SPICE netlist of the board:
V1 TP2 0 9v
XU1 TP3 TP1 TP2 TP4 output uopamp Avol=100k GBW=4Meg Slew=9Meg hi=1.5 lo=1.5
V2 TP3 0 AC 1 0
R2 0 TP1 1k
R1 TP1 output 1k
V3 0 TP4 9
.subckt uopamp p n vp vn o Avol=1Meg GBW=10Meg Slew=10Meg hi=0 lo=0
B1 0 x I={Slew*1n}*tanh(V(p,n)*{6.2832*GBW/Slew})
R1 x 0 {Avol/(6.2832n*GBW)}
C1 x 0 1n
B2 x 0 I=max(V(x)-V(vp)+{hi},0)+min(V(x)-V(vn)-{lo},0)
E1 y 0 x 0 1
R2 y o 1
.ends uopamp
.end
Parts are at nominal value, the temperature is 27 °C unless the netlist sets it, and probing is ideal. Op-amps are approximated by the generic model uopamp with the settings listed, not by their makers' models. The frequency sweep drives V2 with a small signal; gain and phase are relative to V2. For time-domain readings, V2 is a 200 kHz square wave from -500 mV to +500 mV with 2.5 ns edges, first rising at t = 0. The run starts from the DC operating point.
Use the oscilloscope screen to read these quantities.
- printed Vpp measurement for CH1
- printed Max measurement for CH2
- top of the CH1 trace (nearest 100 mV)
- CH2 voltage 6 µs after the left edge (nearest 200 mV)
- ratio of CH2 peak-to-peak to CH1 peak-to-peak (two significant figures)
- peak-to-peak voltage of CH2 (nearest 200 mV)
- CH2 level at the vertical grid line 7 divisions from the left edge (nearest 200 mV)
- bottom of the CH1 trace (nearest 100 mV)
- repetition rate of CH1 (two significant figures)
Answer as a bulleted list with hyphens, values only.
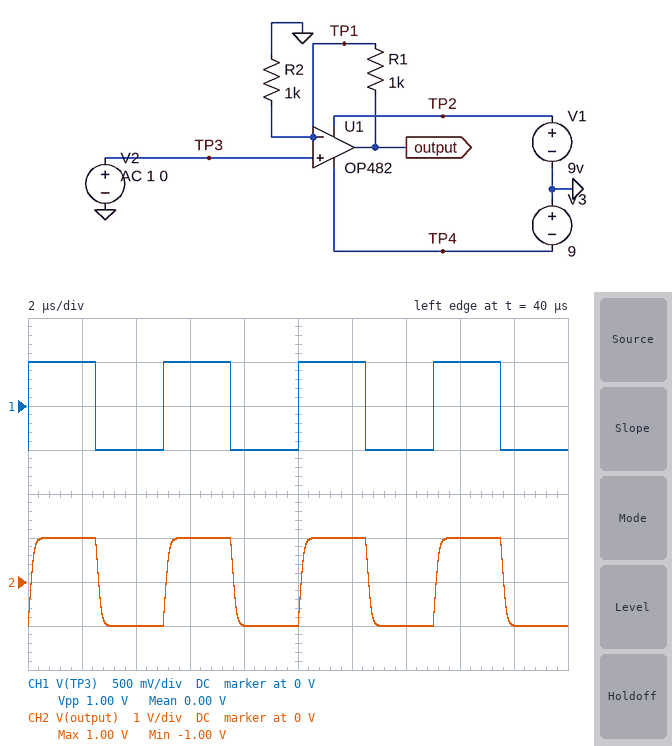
- 1.00 V
- 1.00 V
- 500 mV
- 1.0 V
- 2.0
- 2.0 V
- -1.0 V
- -500 mV
- 200 kHz
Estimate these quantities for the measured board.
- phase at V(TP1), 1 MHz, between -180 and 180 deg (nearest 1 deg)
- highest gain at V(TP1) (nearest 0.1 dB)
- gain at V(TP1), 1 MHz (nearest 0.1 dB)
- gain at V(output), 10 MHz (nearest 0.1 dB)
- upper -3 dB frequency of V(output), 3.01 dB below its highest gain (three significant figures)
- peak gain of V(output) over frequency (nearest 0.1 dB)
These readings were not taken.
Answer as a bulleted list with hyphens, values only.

- -27 deg
- 0 dB
- -1.0 dB
- -8.1 dB
- 2.00 MHz
- 6.0 dB
